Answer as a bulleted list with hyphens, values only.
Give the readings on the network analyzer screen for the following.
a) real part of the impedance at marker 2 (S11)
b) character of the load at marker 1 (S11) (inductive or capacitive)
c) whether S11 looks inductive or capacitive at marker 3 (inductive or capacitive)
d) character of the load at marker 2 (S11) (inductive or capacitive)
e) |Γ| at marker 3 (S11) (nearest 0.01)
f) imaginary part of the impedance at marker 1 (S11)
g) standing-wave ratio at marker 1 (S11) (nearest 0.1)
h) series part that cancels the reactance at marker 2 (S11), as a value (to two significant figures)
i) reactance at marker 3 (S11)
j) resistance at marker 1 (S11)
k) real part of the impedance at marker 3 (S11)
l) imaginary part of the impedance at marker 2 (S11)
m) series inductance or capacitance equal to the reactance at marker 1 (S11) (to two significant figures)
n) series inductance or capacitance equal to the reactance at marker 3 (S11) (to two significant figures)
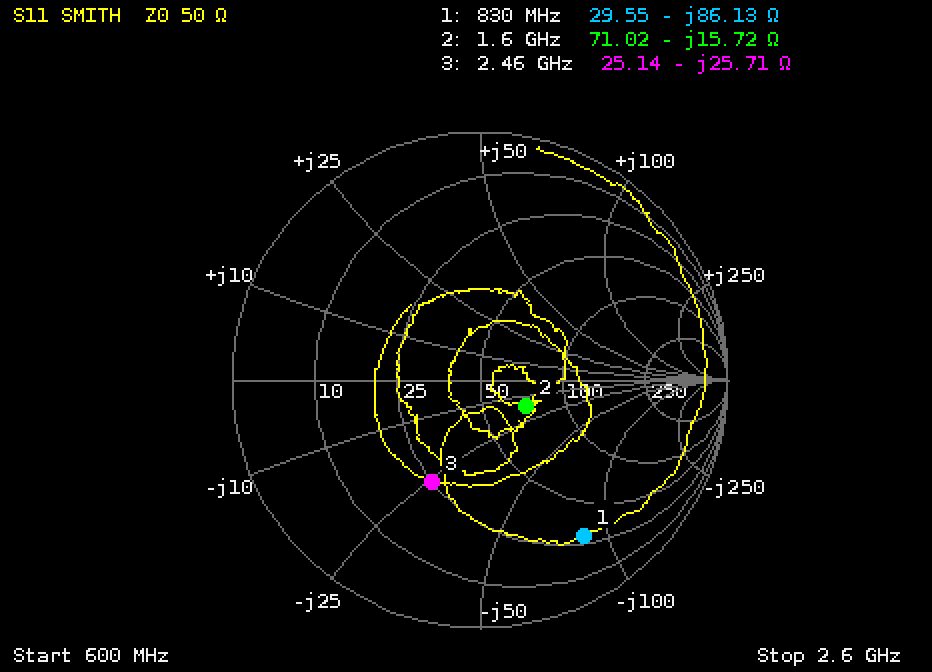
- 71.02 Ω
- capacitive
- capacitive
- capacitive
- 0.45
- -86.13 Ω
- 7.2
- 1.6 nH
- -25.71 Ω
- 29.55 Ω
- 25.14 Ω
- -15.72 Ω
- 2.2 pF
- 2.5 pF
